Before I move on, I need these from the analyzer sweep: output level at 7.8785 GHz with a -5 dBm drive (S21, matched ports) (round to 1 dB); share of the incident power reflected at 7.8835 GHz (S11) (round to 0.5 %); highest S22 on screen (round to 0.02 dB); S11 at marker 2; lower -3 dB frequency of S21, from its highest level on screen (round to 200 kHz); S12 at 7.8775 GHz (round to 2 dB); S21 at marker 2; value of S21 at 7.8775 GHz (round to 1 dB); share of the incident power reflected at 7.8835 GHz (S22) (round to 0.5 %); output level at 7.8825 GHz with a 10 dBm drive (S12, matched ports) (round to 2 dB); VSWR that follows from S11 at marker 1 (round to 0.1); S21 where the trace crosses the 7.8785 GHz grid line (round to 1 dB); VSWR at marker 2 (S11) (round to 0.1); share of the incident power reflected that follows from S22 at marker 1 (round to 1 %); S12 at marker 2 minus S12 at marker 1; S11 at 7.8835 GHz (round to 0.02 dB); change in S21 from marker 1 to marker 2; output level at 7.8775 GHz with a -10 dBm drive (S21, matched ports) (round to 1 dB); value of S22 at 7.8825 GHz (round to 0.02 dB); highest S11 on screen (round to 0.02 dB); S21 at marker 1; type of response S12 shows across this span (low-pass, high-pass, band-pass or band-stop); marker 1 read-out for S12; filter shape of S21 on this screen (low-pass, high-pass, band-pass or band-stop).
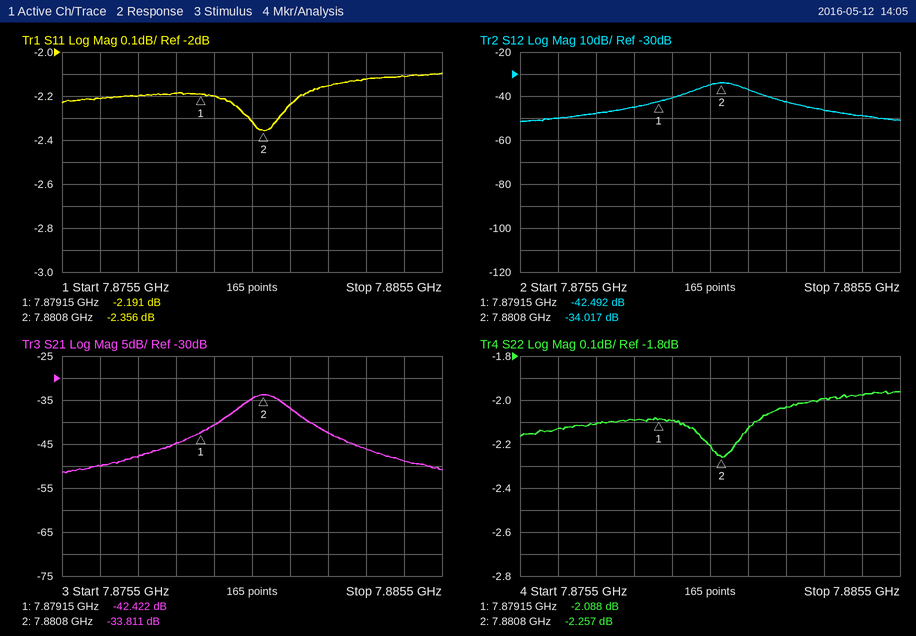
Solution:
-50 dBm
61.5 %
-1.96 dB
-2.356 dB
7.8802 GHz
-48 dB
-33.811 dB
-48 dB
63.0 %
-32 dBm
8.0
-45 dB
7.4
62 %
8.475 dB
-2.12 dB
8.611 dB
-58 dBm
-2.04 dB
-2.10 dB
-42.422 dB
band-pass
-42.492 dB
band-pass
